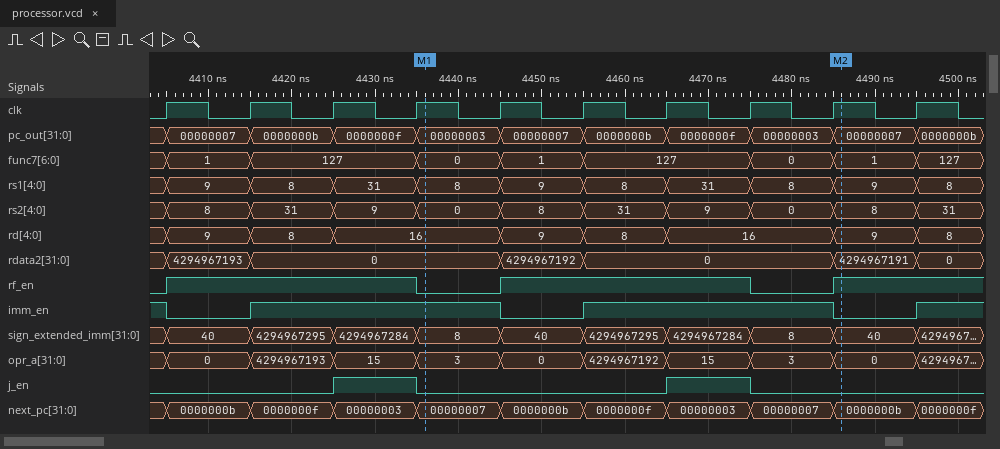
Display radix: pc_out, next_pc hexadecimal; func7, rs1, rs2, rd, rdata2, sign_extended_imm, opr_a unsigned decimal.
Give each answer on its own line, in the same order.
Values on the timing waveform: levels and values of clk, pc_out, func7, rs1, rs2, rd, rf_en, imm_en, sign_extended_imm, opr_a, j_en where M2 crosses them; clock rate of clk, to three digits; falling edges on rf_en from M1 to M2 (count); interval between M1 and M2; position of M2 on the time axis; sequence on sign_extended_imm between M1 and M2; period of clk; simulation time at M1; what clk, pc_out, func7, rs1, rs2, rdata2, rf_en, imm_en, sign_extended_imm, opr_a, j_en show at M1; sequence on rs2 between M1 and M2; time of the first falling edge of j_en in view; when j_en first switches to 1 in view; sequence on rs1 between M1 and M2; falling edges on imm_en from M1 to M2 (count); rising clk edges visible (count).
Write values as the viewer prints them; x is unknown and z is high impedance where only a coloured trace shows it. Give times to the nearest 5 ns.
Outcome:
clk=1, pc_out=00000007, func7=1, rs1=9, rs2=8, rd=9, rf_en=1, imm_en=0, sign_extended_imm=40, opr_a=0, j_en=0
100 MHz
1
50 ns
4485 ns
8, 40, 4294967295, 4294967284, 8, 40
10 ns
4435 ns
clk=1, pc_out=00000003, func7=0, rs1=8, rs2=0, rdata2=0, rf_en=0, imm_en=1, sign_extended_imm=8, opr_a=3, j_en=0
0, 8, 31, 9, 0, 8
4435 ns
4425 ns
8, 9, 8, 31, 8, 9
2
10
